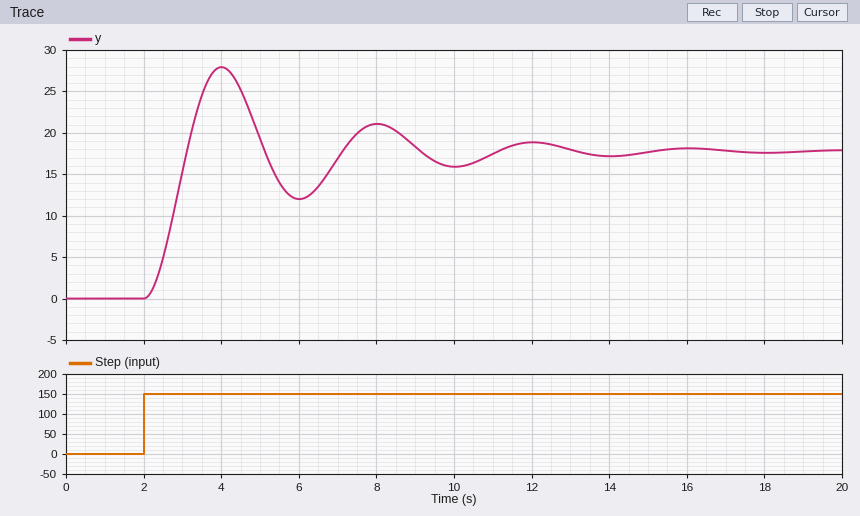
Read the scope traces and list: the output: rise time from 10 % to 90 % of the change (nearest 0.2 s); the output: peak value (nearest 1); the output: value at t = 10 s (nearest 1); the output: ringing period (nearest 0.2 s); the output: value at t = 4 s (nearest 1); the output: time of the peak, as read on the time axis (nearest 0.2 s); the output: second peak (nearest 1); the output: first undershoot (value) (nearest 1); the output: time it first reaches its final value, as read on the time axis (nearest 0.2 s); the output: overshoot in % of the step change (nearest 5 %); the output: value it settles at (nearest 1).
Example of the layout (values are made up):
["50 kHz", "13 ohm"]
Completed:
["0.8 s", "28", "16", "4.0 s", "28", "4.0 s", "21", "12", "3.2 s", "55 %", "18"]
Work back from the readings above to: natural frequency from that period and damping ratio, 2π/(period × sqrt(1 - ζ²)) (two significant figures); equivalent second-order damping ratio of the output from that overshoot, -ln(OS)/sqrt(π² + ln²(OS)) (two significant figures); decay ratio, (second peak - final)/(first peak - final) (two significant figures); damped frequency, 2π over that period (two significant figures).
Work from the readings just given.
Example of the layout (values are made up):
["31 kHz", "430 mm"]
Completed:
["1.6 rad/s", "0.19", "0.30", "1.6 rad/s"]
